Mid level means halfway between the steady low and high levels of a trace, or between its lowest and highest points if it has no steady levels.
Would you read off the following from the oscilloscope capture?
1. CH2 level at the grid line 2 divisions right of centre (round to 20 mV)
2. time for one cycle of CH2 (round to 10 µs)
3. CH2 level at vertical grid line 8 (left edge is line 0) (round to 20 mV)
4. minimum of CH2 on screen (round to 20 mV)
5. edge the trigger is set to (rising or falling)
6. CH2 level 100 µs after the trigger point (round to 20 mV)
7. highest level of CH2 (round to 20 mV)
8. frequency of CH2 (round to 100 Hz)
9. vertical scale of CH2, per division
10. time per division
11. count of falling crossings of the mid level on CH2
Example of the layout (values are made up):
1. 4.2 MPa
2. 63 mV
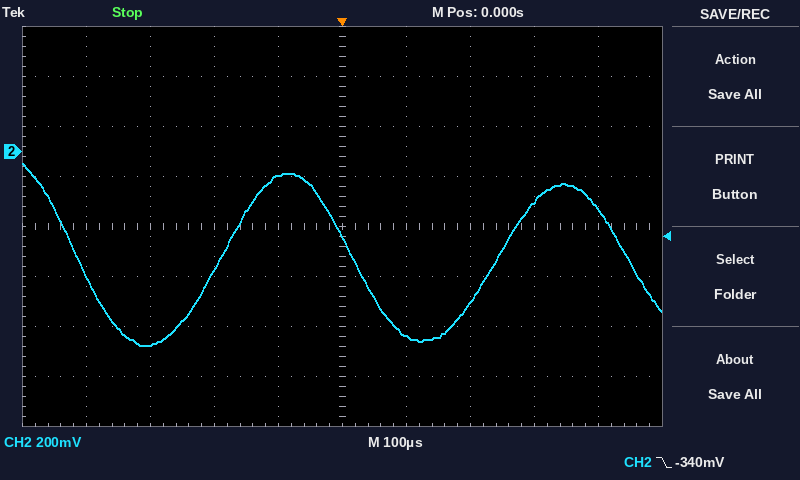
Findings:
1. -600 mV
2. 430 µs
3. -200 mV
4. -780 mV
5. falling
6. -740 mV
7. -40 mV
8. 2.3 kHz
9. 200 mV
10. 100 µs
11. 3
